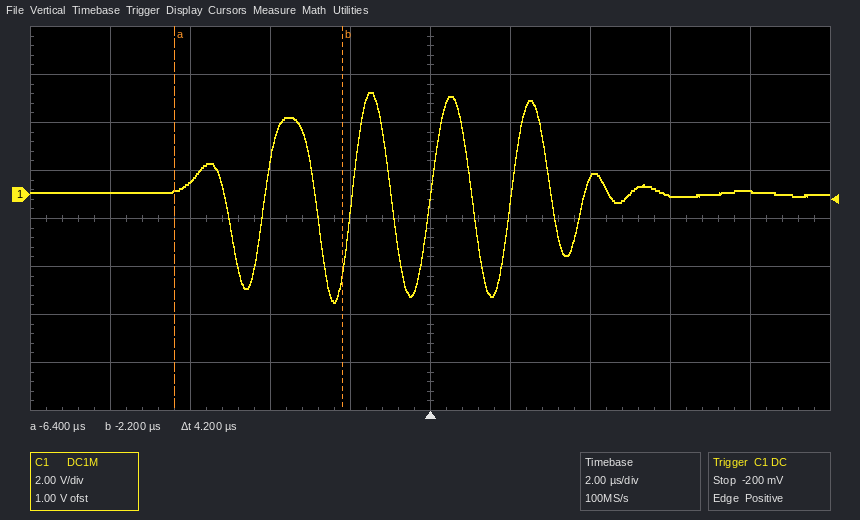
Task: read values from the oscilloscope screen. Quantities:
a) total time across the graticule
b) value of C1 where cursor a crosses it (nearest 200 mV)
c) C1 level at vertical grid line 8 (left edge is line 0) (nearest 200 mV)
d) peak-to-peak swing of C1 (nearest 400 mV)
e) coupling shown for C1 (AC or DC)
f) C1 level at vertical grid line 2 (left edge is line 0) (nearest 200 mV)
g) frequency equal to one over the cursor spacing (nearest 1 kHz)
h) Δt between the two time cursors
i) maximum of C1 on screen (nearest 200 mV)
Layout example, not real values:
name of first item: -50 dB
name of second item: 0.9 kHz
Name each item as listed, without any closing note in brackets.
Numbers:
total time across the graticule: 20 µs
value of C1 where cursor a crosses it: 200 mV
C1 level at vertical grid line 8 (left edge is line 0): 0.0 V
peak-to-peak swing of C1: 8.8 V
coupling shown for C1: DC
C1 level at vertical grid line 2 (left edge is line 0): 600 mV
frequency equal to one over the cursor spacing: 238 kHz
Δt between the two time cursors: 4.2 µs
maximum of C1 on screen: 4.2 V
